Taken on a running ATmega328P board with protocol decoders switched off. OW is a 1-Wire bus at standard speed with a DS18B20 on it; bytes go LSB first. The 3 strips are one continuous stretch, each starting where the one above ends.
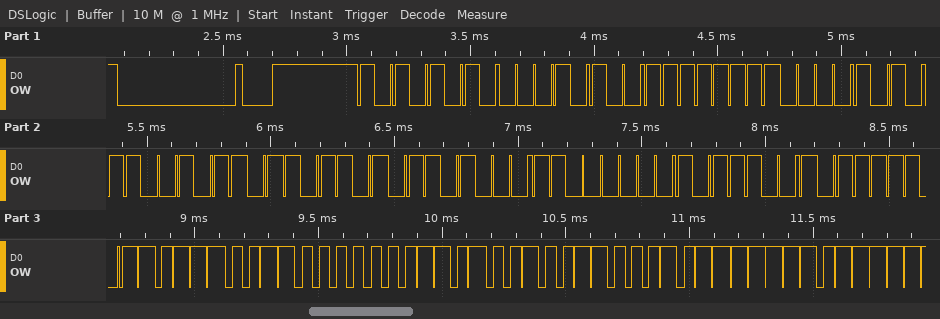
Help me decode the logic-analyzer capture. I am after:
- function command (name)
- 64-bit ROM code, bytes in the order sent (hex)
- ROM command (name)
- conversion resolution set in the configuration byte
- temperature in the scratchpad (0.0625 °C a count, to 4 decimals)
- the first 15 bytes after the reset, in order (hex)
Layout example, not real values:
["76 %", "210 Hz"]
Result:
["Read Scratchpad", "28 FF 50 D3 B6 16 03 9D", "Match ROM", "12 bits", "25.8125 °C", "55 28 FF 50 D3 B6 16 03 9D BE 9D 01 4B 46 7F"]
